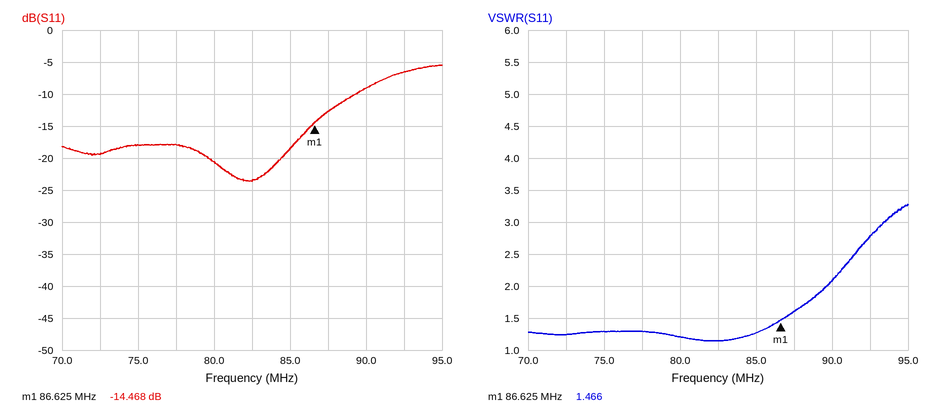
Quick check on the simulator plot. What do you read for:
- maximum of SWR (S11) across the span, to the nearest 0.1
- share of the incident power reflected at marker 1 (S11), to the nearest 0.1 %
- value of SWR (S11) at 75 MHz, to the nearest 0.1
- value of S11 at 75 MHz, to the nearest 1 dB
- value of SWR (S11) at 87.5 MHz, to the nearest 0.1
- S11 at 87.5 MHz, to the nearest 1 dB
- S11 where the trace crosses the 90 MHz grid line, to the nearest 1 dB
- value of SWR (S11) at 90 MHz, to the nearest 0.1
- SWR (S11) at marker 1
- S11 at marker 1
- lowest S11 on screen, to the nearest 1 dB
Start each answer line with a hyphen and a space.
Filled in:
- 3.3
- 3.6 %
- 1.3
- -18 dB
- 1.6
- -13 dB
- -9 dB
- 2.1
- 1.466
- -14.468 dB
- -24 dB
